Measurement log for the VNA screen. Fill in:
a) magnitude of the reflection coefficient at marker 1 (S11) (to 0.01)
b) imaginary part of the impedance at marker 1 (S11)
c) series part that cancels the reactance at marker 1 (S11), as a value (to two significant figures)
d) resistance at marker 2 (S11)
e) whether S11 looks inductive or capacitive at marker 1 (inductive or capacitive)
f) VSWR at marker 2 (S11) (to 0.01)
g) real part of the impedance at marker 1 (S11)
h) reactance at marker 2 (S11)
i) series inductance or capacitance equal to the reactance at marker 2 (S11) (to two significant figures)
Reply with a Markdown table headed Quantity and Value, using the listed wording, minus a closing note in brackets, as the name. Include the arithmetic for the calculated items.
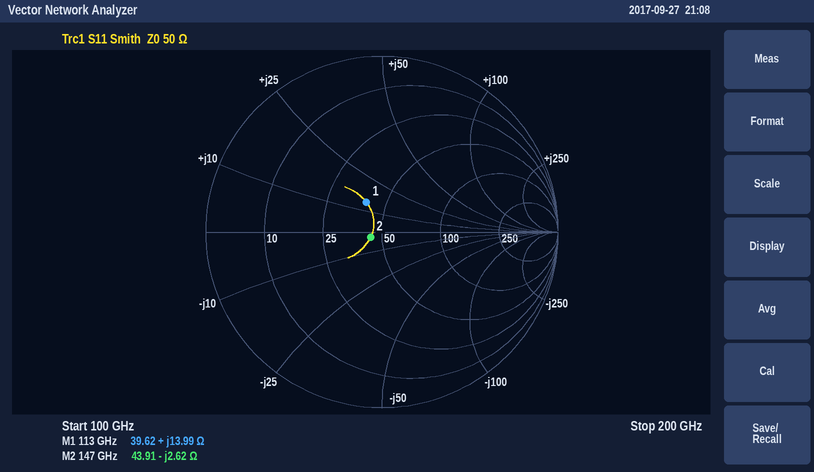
| Quantity | Value |
|---|---|
| magnitude of the reflection coefficient at marker 1 (S11) | 0.19 |
| imaginary part of the impedance at marker 1 | +13.99 Ω |
| series part that cancels the reactance at marker 1 (S11), as a value | C = 1/(2π × 113 GHz × 13.99 Ω) ≈ 101 fF, so 100 fF to two significant figures |
| resistance at marker 2 | 43.91 Ω |
| whether S11 looks inductive or capacitive at marker 1 | inductive |
| VSWR at marker 2 (S11) | 1.15 |
| real part of the impedance at marker 1 | 39.62 Ω |
| reactance at marker 2 | -2.62 Ω |
| series inductance or capacitance equal to the reactance at marker 2 (S11) | C = 1/(2π × 147 GHz × 2.62 Ω) ≈ 413 fF, so 410 fF to two significant figures |
